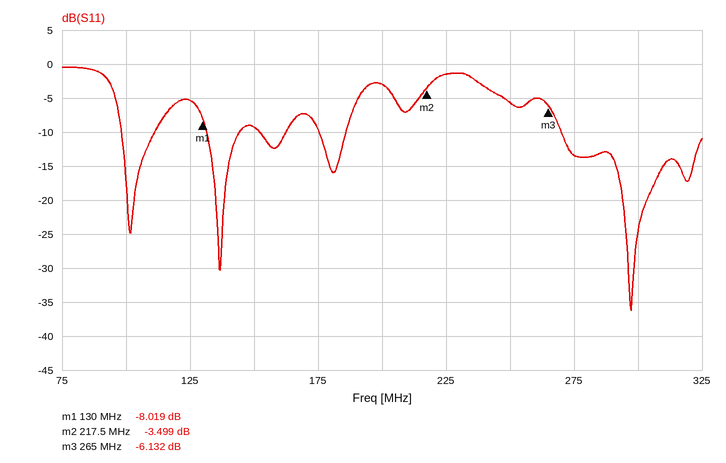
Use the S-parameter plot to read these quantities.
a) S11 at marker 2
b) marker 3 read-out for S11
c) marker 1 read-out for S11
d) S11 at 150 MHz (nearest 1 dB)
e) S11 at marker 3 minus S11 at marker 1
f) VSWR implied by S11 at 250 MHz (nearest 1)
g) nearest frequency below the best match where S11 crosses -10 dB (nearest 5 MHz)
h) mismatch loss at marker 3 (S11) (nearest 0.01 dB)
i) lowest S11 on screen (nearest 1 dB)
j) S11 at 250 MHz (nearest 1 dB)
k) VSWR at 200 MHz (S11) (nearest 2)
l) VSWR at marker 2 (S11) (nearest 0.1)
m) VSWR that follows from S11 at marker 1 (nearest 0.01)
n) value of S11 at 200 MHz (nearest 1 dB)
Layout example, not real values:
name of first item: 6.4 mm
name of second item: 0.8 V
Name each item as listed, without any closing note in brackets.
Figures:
S11 at marker 2: -3.499 dB
marker 3 read-out for S11: -6.132 dB
marker 1 read-out for S11: -8.019 dB
S11 at 150 MHz: -9 dB
S11 at marker 3 minus S11 at marker 1: 1.887 dB
VSWR implied by S11 at 250 MHz: 3
nearest frequency below the best match where S11 crosses -10 dB: 270 MHz
mismatch loss at marker 3 (S11): 1.21 dB
lowest S11 on screen: -36 dB
S11 at 250 MHz: -6 dB
VSWR at 200 MHz (S11): 6
VSWR at marker 2 (S11): 5.0
VSWR that follows from S11 at marker 1: 2.32
value of S11 at 200 MHz: -3 dB
